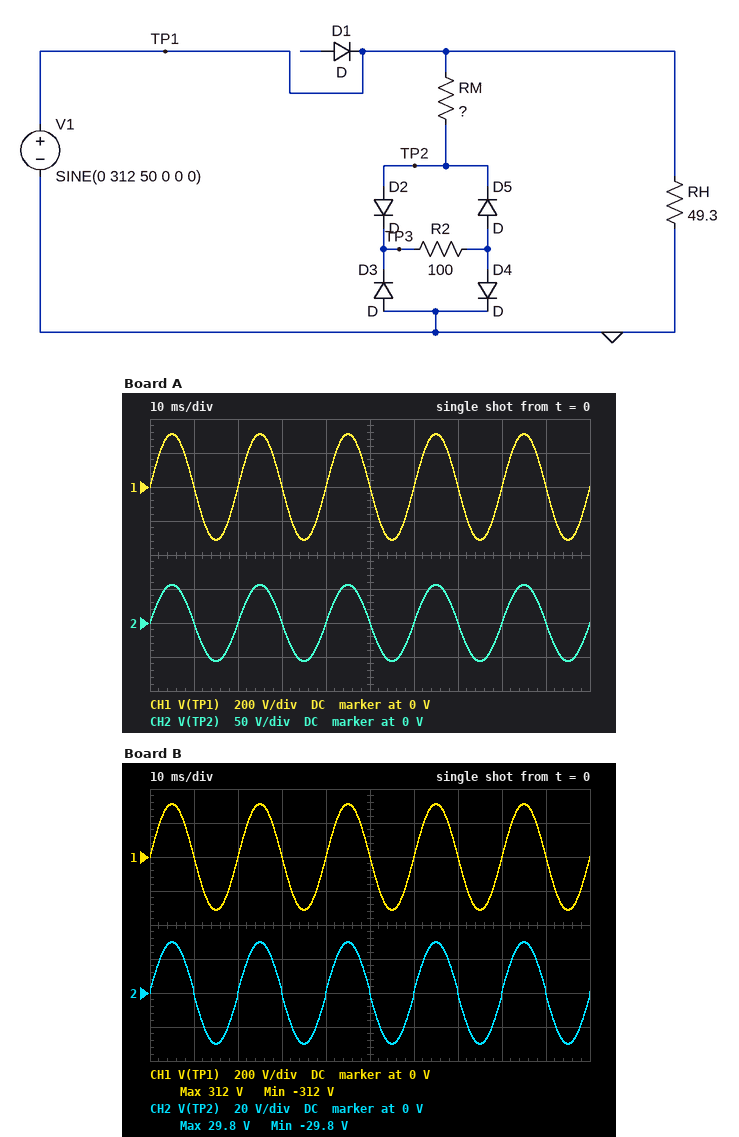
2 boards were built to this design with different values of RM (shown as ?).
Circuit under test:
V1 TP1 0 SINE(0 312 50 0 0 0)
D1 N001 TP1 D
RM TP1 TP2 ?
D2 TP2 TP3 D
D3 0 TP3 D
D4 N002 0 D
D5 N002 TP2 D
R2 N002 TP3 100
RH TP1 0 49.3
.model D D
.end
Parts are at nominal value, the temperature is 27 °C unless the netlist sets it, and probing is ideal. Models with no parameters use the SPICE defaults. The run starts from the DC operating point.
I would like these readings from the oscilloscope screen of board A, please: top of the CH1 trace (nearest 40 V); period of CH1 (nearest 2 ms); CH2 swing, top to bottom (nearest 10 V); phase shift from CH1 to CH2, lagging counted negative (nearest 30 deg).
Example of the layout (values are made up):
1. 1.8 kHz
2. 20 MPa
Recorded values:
1. 320 V
2. 20 ms
3. 110 V
4. 0 deg
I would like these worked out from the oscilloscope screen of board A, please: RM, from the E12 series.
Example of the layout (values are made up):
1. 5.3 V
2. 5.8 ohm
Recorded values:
1. 470 Ω
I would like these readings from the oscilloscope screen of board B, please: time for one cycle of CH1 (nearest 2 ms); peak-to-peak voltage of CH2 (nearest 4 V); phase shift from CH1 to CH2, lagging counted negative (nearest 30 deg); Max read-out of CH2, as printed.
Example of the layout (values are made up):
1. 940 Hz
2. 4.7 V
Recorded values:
1. 20 ms
2. 60 V
3. 0 deg
4. 29.8 V
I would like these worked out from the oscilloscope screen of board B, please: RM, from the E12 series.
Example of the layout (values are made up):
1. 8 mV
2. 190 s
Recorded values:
1. 1 kΩ
